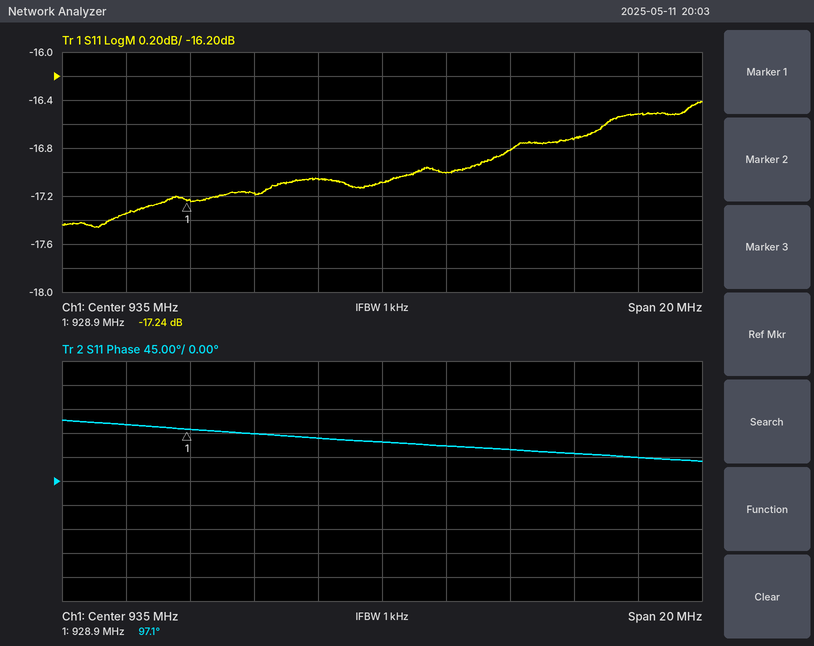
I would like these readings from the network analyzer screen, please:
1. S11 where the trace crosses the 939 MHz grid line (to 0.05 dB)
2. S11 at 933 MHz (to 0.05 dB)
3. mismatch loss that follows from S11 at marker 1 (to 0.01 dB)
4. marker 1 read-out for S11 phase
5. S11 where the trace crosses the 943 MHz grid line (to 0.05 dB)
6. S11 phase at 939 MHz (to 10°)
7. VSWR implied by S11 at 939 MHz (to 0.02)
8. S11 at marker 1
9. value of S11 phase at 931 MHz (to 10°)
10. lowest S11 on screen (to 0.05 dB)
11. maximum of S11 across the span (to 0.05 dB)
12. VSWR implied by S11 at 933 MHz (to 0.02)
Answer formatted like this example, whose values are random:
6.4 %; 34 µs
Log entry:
-16.80 dB; -17.05 dB; 0.08 dB; 97.1°; -16.50 dB; 60°; 1.34; -17.24 dB; 90°; -17.45 dB; -16.40 dB; 1.32
